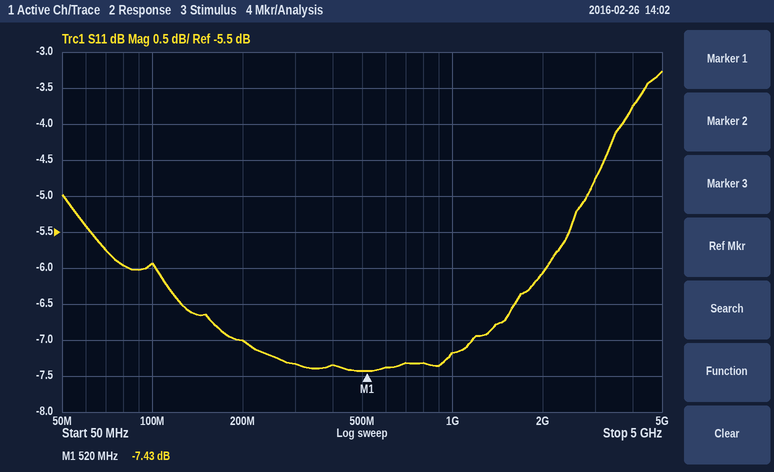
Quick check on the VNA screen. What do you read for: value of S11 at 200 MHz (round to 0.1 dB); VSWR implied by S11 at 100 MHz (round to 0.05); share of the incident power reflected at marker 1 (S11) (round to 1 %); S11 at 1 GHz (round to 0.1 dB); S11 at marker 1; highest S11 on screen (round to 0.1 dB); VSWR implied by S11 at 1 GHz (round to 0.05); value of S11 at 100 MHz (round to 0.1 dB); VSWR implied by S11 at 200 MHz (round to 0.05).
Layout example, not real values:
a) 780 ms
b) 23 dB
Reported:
a) -7.0 dB
b) 3.05
c) 18 %
d) -7.2 dB
e) -7.43 dB
f) -3.3 dB
g) 2.55
h) -5.9 dB
i) 2.60
